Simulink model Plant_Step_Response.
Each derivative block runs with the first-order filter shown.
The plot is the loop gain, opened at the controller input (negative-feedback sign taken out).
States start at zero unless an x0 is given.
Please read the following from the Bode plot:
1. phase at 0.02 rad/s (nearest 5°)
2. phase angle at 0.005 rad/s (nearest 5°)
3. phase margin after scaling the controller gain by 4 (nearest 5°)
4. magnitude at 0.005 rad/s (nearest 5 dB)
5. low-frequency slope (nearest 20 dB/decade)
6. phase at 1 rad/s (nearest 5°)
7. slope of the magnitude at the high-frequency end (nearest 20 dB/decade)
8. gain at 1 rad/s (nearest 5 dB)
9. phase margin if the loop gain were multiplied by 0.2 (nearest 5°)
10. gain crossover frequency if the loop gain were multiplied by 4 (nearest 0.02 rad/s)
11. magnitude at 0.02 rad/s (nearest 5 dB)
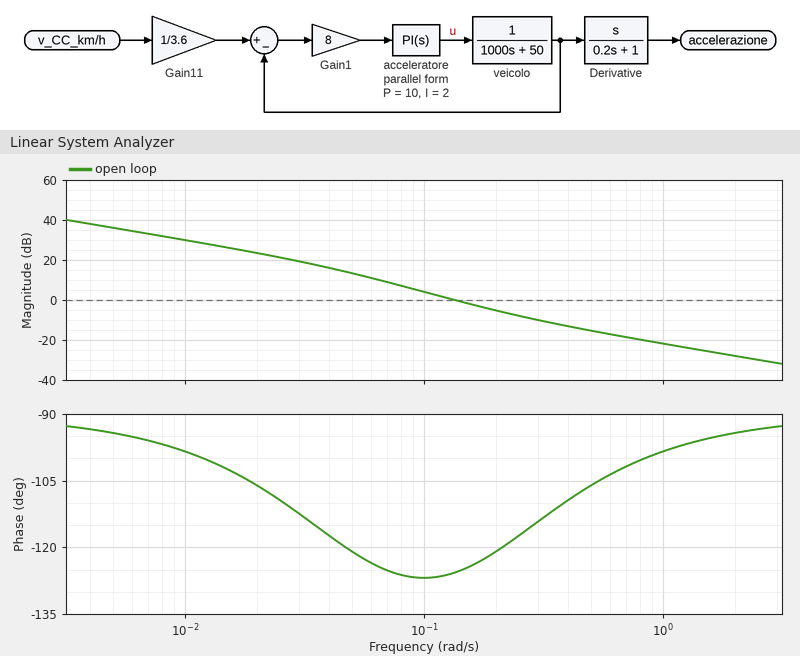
-105°
-95°
70°
35 dB
-20 dB/decade
-100°
-20 dB/decade
-20 dB
60°
0.36 rad/s
25 dB
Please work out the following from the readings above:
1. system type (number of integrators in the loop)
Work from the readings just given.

1
